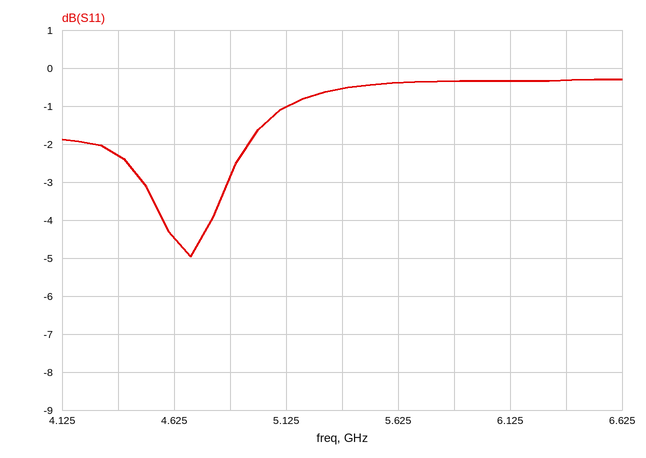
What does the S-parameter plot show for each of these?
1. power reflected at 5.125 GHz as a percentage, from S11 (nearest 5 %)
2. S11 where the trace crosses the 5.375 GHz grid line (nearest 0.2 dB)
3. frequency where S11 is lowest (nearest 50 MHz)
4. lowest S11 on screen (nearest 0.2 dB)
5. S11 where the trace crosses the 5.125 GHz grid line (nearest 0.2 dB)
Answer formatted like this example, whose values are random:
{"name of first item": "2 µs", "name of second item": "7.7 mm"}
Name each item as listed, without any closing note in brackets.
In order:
{"power reflected at 5.125 GHz as a percentage, from S11": "80 %", "S11 where the trace crosses the 5.375 GHz grid line": "-0.6 dB", "frequency where S11 is lowest": "4.70 GHz", "lowest S11 on screen": "-5.0 dB", "S11 where the trace crosses the 5.125 GHz grid line": "-1.0 dB"}
